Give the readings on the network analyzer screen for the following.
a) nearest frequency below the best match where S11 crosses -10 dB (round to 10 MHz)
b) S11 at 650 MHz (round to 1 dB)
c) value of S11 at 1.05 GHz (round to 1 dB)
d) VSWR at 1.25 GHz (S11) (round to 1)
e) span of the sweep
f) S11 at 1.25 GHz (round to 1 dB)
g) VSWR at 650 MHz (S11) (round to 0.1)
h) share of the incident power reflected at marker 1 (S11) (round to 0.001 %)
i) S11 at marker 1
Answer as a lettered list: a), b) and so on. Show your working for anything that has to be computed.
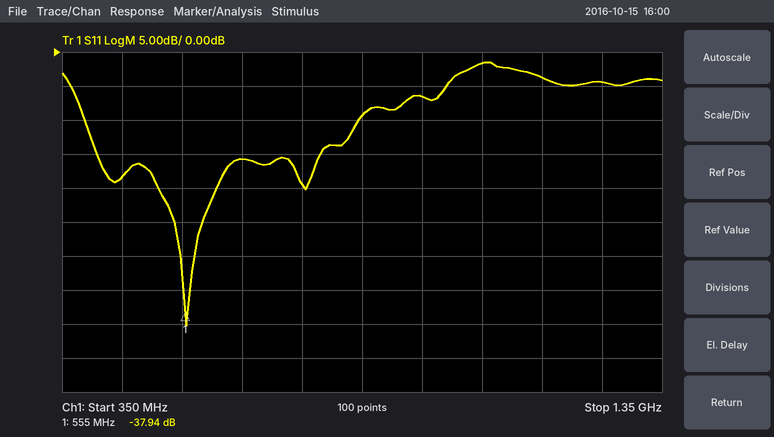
a) 390 MHz
b) -16 dB
c) -2 dB
d) |Γ| = 10^(-4/20) = 0.6310; VSWR = (1 + 0.6310)/(1 − 0.6310) ≈ 4
e) 1 GHz
f) -4 dB
g) |Γ| = 10^(-16/20) = 0.1585; VSWR = (1 + 0.1585)/(1 − 0.1585) ≈ 1.4
h) 10^(-37.94/10) ≈ 0.016 %
i) -37.94 dB
